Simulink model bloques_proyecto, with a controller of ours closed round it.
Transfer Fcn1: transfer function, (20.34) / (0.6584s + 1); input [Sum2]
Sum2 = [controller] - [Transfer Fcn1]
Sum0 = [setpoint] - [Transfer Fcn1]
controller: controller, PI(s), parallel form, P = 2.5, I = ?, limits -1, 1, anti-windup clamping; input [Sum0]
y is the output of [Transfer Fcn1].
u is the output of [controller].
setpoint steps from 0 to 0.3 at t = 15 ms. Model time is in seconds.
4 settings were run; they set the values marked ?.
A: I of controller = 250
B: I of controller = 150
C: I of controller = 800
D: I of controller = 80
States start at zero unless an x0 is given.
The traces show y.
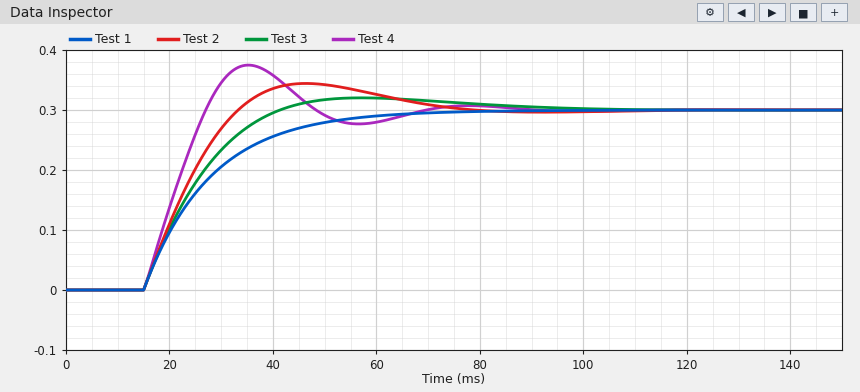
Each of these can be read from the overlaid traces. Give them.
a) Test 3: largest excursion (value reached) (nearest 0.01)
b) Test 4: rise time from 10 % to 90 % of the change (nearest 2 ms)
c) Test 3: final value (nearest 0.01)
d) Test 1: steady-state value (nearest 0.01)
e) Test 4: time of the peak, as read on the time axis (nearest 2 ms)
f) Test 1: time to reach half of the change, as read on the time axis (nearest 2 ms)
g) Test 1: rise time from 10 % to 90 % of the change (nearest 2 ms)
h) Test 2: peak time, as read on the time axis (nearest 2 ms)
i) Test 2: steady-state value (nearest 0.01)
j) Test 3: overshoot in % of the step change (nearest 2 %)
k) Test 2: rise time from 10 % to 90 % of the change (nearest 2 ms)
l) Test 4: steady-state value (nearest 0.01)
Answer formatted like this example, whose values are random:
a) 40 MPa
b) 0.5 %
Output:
a) 0.32
b) 10 ms
c) 0.30
d) 0.30
e) 36 ms
f) 24 ms
g) 28 ms
h) 46 ms
i) 0.30
j) 6 %
k) 14 ms
l) 0.30
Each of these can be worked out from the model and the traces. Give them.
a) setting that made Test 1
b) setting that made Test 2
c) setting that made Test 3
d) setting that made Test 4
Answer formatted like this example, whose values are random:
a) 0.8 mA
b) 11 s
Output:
a) D
b) A
c) B
d) C
